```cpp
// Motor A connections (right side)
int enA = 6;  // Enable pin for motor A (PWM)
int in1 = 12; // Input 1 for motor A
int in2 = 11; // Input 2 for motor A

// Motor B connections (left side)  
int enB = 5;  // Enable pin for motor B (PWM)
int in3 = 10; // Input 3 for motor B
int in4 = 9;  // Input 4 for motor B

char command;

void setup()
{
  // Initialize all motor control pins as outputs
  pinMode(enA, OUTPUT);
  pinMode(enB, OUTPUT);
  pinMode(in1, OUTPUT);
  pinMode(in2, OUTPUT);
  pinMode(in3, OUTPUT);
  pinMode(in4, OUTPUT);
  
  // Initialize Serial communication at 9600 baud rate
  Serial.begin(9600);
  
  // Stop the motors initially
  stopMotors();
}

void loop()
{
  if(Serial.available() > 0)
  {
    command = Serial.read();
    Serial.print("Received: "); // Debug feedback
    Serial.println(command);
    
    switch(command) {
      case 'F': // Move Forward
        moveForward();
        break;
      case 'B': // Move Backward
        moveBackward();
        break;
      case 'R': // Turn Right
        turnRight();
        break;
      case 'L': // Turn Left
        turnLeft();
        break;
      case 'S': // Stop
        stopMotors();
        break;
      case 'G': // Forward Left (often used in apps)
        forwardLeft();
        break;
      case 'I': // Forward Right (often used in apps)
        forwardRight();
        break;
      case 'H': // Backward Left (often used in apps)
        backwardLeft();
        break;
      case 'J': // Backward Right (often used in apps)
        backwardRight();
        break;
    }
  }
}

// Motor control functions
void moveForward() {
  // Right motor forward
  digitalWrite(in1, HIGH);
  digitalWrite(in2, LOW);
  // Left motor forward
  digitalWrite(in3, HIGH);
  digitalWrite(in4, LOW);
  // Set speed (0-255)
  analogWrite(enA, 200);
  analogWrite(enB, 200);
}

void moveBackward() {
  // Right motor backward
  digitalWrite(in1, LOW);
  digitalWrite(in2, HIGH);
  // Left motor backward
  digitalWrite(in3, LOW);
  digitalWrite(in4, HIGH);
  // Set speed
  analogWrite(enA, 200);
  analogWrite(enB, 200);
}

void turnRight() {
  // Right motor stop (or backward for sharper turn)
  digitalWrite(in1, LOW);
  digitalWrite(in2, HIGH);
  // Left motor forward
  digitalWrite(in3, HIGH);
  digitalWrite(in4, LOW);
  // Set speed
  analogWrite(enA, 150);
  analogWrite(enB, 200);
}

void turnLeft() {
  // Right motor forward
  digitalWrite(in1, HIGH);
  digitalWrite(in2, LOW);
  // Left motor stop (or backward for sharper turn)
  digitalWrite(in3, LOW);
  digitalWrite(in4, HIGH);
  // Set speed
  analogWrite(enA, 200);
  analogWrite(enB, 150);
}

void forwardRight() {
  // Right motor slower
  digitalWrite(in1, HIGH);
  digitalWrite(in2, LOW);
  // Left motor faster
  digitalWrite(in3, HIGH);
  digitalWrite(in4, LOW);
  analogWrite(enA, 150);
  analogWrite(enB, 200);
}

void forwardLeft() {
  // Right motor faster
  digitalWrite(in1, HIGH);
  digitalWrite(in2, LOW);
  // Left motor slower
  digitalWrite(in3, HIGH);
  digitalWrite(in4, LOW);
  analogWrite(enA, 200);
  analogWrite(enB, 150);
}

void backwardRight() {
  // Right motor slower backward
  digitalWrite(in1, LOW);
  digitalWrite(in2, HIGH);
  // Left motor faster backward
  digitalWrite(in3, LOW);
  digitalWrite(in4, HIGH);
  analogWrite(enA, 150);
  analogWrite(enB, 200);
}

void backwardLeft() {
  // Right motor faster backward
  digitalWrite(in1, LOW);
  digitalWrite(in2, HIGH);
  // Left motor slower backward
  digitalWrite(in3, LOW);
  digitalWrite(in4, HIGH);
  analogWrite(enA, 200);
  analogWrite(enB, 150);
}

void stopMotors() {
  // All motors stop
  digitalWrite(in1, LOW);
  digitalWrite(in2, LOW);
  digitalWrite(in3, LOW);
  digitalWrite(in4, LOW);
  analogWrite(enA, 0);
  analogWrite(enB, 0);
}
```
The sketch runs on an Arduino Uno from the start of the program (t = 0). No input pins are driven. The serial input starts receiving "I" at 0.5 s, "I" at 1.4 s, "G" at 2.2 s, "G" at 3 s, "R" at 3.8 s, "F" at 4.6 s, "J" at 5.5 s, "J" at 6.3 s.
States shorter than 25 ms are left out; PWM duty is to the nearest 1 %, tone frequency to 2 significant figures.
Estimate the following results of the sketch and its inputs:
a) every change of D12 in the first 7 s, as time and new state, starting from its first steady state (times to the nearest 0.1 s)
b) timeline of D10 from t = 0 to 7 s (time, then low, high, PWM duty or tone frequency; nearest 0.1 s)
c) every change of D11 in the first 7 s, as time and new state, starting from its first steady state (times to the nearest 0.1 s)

0 s low; 0.5 s high; 3.8 s low; 4.6 s high; 5.5 s low
0 s low; 0.5 s high; 5.5 s low
0 s low; 3.8 s high; 4.6 s low; 5.5 s high
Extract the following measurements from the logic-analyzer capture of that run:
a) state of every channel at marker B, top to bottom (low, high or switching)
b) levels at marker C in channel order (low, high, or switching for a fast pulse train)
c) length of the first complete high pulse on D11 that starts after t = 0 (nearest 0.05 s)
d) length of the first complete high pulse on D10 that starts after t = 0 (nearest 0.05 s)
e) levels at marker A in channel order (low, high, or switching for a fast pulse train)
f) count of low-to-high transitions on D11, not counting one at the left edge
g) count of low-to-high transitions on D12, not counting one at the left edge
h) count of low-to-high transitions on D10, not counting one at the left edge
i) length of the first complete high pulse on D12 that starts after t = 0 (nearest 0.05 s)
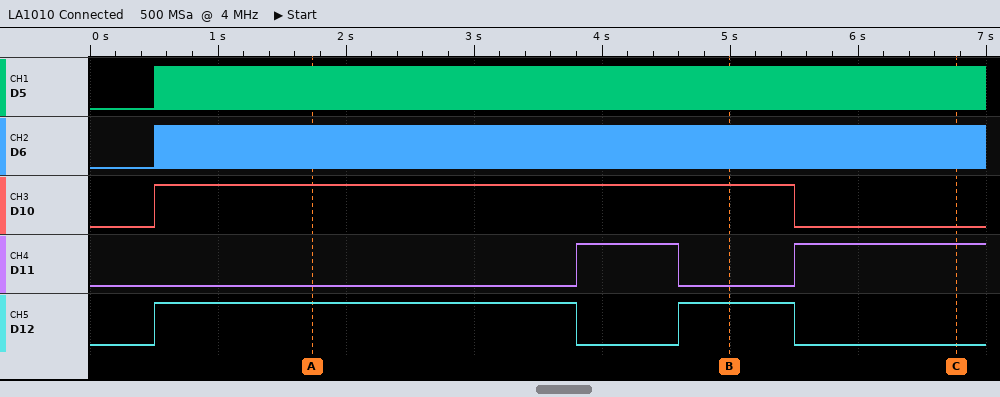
D5 switching, D6 switching, D10 high, D11 low, D12 high
D5 switching, D6 switching, D10 low, D11 high, D12 low
0.80 s
5.00 s
D5 switching, D6 switching, D10 high, D11 low, D12 high
2
2
1
3.30 s
